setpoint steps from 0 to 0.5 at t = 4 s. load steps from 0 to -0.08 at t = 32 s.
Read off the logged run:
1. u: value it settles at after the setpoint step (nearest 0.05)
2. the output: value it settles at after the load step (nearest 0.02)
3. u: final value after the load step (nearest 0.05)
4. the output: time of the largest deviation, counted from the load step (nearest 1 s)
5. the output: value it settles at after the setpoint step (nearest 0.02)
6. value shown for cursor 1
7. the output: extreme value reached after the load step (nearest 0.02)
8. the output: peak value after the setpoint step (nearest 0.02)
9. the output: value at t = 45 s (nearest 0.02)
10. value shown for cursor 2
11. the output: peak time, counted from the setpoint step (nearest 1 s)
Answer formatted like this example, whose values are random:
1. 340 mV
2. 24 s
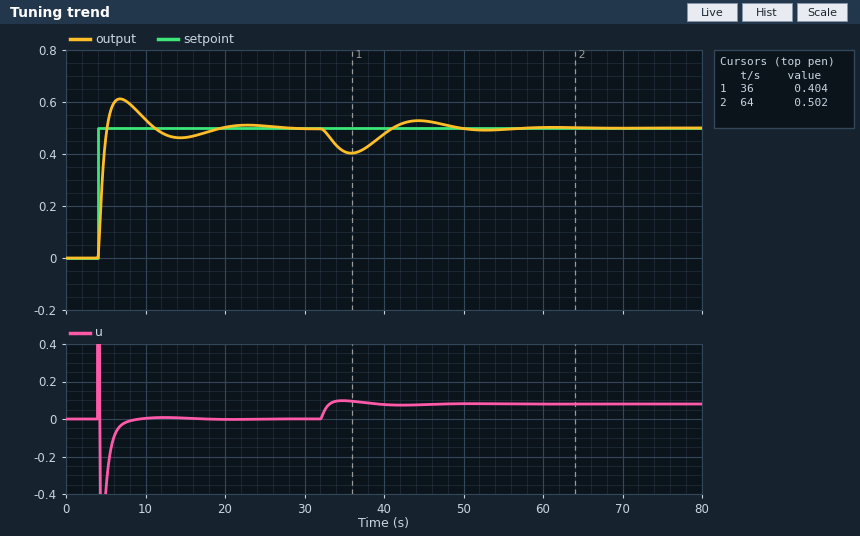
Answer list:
1. 0.00
2. 0.50
3. 0.10
4. 4 s
5. 0.50
6. 0.404
7. 0.40
8. 0.62
9. 0.52
10. 0.502
11. 3 s
